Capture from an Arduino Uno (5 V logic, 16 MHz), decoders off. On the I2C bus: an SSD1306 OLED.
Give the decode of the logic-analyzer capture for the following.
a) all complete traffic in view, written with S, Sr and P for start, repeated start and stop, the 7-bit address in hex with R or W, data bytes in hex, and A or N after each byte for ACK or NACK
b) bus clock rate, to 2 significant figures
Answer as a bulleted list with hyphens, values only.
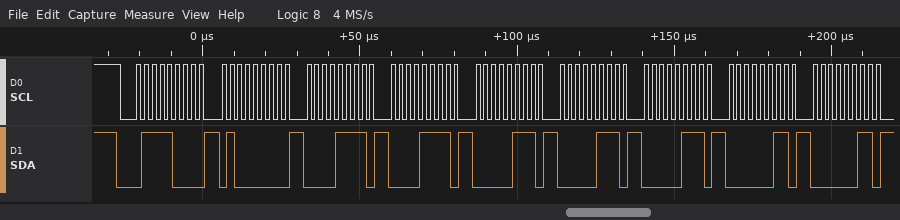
- S 3CW A 40 A 0F A 0F A 07 A 07 A 07 A 03 A 03 A
- 400 kHz
